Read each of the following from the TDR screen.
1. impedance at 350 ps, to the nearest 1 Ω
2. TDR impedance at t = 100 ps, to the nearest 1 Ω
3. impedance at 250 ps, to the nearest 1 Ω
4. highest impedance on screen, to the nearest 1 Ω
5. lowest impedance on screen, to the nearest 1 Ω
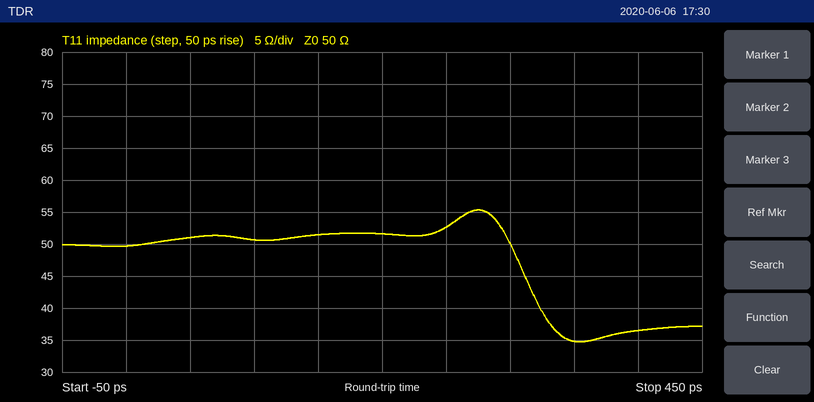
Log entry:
35 Ω
51 Ω
53 Ω
55 Ω
35 Ω
